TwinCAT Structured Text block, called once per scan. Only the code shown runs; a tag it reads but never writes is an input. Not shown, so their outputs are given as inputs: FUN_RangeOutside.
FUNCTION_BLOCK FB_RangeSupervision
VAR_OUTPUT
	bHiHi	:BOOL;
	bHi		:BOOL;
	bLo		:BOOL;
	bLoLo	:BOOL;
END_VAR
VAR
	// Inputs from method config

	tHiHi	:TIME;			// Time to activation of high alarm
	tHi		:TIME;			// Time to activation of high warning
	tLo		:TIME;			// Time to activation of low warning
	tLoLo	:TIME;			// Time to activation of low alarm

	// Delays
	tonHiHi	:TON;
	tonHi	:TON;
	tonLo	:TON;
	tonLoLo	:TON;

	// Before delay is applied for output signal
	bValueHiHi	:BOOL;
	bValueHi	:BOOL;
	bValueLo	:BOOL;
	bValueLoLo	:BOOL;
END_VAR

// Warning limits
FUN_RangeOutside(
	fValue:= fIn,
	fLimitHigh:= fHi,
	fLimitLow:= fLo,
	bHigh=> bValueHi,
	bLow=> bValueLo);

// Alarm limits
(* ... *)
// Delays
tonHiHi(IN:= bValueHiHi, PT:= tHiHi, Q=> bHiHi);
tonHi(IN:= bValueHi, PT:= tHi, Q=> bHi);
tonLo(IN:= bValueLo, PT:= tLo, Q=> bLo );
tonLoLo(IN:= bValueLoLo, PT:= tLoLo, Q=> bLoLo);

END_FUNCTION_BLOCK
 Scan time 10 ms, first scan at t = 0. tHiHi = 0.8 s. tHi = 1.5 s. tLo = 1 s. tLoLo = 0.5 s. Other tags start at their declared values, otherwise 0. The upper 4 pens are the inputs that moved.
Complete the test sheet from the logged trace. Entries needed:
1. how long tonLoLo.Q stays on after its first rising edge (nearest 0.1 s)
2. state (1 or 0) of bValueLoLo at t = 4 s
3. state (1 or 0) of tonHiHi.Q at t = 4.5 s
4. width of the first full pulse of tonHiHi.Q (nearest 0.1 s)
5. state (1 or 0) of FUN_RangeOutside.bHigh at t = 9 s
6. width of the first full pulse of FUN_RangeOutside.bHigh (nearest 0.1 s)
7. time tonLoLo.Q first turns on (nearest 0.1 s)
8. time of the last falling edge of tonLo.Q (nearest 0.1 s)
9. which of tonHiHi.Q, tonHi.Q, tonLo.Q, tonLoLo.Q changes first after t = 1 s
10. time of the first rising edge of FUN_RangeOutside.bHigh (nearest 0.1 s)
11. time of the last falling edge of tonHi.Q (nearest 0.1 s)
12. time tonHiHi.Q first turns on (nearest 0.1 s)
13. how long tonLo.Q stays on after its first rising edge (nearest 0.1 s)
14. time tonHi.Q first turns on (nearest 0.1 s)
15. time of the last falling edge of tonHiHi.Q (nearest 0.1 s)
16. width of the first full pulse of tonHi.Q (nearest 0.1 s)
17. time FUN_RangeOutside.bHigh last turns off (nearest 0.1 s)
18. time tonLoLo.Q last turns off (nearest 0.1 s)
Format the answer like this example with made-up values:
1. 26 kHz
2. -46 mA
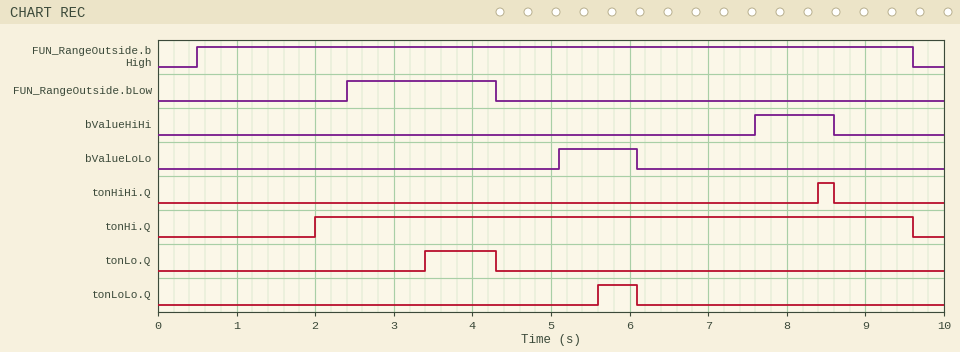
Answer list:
1. 0.5 s
2. 0
3. 0
4. 0.2 s
5. 1
6. 9.1 s
7. 5.6 s
8. 4.3 s
9. tonHi.Q
10. 0.5 s
11. 9.6 s
12. 8.4 s
13. 0.9 s
14. 2.0 s
15. 8.6 s
16. 7.6 s
17. 9.6 s
18. 6.1 s
